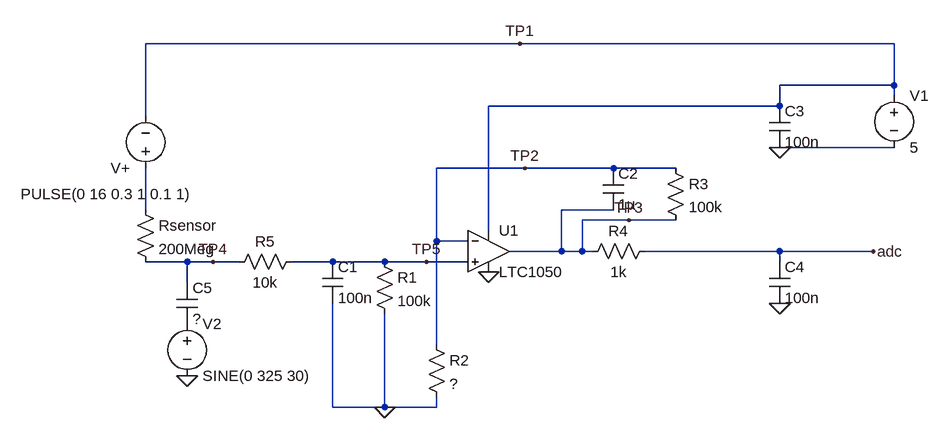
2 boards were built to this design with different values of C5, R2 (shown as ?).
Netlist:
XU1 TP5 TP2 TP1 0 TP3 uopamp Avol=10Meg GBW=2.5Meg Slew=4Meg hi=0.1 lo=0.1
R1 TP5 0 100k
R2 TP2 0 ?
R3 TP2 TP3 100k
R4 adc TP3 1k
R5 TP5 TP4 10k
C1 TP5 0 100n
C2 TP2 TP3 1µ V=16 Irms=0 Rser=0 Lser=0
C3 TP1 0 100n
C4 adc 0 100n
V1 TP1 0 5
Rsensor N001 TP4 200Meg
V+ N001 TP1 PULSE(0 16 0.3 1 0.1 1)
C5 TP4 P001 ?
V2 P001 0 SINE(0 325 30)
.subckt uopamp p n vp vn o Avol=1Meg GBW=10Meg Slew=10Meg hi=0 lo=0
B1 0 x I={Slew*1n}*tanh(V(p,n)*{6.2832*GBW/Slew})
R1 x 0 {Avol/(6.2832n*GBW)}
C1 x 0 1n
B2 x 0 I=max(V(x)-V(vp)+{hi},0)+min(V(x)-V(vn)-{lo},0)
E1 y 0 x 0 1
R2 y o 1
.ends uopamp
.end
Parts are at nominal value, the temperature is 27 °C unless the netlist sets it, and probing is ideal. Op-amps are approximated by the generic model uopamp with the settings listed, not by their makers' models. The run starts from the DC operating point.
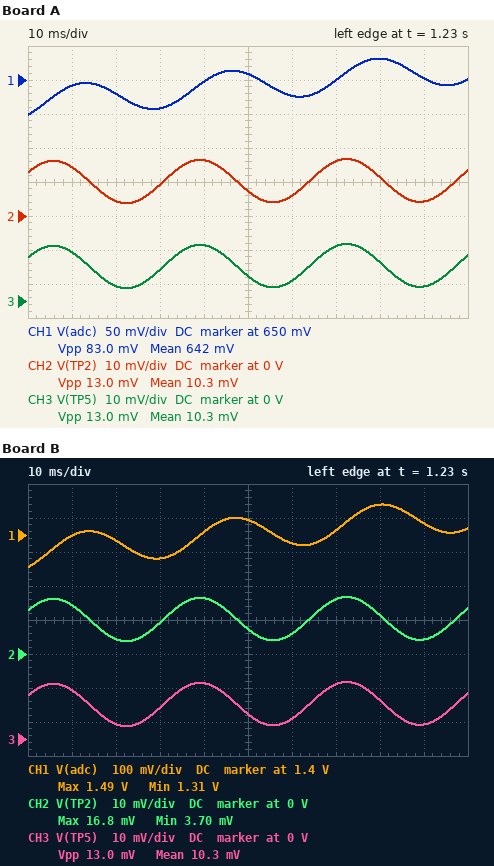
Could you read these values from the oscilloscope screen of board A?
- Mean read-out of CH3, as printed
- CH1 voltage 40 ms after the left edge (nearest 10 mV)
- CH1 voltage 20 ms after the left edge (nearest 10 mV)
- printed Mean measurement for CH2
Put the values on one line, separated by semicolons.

10.3 mV; 650 mV; 630 mV; 10.3 mV
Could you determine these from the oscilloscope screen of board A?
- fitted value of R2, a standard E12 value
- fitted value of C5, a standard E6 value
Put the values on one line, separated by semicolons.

1.5 kΩ; 2.2 pF
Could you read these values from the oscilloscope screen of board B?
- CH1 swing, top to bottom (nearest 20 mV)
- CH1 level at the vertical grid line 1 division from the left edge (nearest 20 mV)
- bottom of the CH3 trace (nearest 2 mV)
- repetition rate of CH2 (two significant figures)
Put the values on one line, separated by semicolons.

180 mV; 1.40 V; 4 mV; 30 Hz
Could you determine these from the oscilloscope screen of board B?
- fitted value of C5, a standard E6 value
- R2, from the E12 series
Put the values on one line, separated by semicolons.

2.2 pF; 680 Ω
